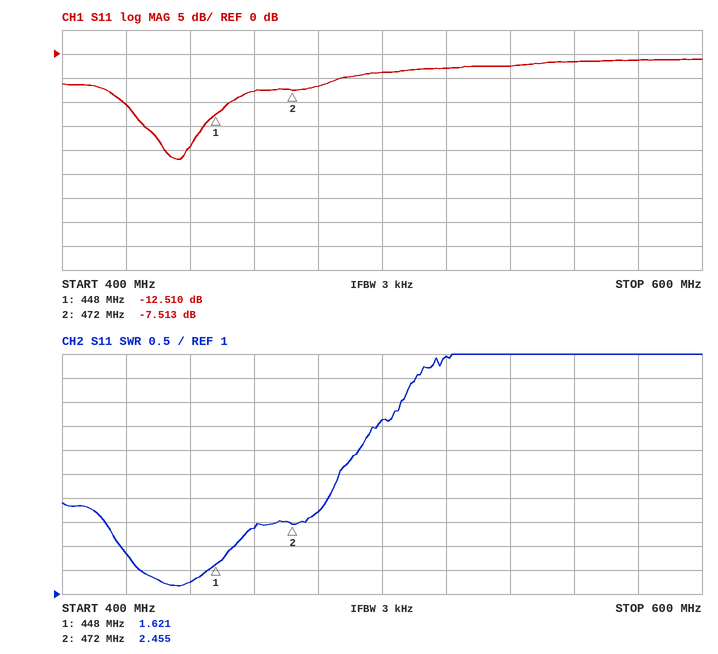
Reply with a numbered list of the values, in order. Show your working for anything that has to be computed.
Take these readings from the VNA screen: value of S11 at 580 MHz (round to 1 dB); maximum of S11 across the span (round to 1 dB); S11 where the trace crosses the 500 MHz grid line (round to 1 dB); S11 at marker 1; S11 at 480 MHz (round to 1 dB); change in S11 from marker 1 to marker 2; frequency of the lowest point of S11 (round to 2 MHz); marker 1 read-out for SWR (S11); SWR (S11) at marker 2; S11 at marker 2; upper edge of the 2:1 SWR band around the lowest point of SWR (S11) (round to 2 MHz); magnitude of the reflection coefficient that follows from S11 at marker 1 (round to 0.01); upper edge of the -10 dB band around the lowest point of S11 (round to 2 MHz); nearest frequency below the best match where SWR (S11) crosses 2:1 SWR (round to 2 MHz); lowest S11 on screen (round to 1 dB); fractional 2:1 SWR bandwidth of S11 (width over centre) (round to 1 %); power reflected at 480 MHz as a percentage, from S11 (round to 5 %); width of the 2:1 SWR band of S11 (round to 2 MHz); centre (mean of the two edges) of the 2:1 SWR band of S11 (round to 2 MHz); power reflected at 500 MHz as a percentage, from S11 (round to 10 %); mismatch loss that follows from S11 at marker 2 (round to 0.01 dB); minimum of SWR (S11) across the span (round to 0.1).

1. -1 dB
2. -1 dB
3. -4 dB
4. -12.510 dB
5. -7 dB
6. -7.513 − (-12.51) = 4.997 dB
7. 436 MHz
8. 1.621
9. 2.455
10. -7.513 dB
11. 454 MHz
12. 10^(-12.51/20) ≈ 0.24
13. 452 MHz
14. 418 MHz
15. -22 dB
16. 36 MHz / 436 MHz ≈ 8 %
17. 10^(-7/10) ≈ 20 %
18. 454 MHz − 418 MHz = 36 MHz
19. 436 MHz
20. 10^(-4/10) ≈ 40 %
21. −10 log10(1 − 10^(-7.513/10)) ≈ 0.85 dB
22. 1.2
